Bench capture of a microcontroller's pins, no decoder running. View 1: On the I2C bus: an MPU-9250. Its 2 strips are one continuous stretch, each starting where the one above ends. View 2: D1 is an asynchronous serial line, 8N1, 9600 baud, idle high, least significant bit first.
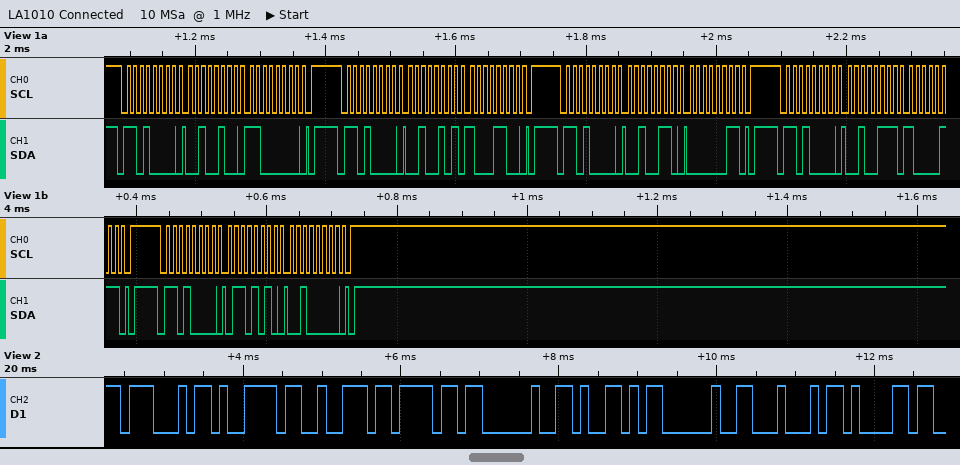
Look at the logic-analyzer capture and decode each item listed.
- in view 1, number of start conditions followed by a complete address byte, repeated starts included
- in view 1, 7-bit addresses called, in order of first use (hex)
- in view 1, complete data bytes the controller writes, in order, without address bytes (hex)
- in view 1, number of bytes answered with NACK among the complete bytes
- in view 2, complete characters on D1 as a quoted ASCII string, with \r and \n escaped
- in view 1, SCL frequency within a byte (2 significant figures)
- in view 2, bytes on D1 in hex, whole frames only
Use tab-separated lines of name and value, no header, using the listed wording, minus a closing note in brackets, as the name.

in view 1, number of start conditions followed by a complete address byte, repeated starts included	5
in view 1, 7-bit addresses called, in order of first use	0x68
in view 1, complete data bytes the controller writes, in order, without address bytes	24 C0 25 8C 26 03 27 87 6A 20
in view 1, number of bytes answered with NACK among the complete bytes	0
in view 2, complete characters on D1 as a quoted ASCII string, with \r and \n escaped	"Gyro Y Da"
in view 1, SCL frequency within a byte	100 kHz
in view 2, bytes on D1 in hex, whole frames only	47 79 72 6F 20 59 20 44 61
